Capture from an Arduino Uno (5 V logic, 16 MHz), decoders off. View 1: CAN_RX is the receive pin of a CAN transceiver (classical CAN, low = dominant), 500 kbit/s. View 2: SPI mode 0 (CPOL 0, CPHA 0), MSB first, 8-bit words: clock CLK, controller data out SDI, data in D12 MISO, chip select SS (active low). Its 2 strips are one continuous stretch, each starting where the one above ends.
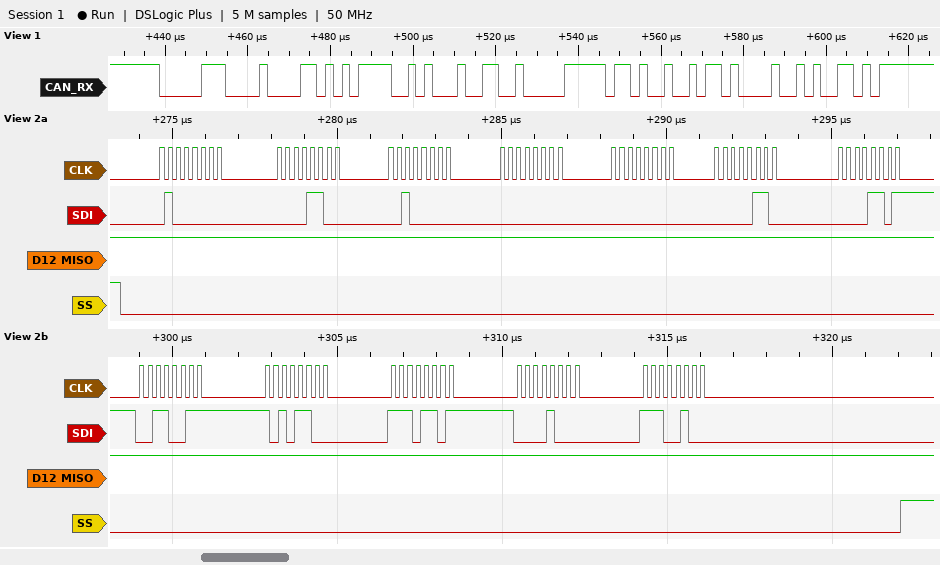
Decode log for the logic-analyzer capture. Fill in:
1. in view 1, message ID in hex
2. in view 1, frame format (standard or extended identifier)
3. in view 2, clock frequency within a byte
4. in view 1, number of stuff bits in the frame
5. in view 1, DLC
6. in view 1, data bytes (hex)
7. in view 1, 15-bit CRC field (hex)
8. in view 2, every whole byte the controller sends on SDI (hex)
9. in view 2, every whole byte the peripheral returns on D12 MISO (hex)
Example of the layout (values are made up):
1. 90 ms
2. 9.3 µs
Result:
1. 0x061
2. standard
3. 4 MHz
4. 3
5. 6
6. AF 28 99 07 E9 2D
7. 0x04A6
8. 0x40 0x0C 0x20 0x00 0x00 0x06 0x0D 0x33 0xAC 0xED 0x08 0xE4
9. 0xFF 0xFF 0xFF 0xFF 0xFF 0xFF 0xFF 0xFF 0xFF 0xFF 0xFF 0xFF
